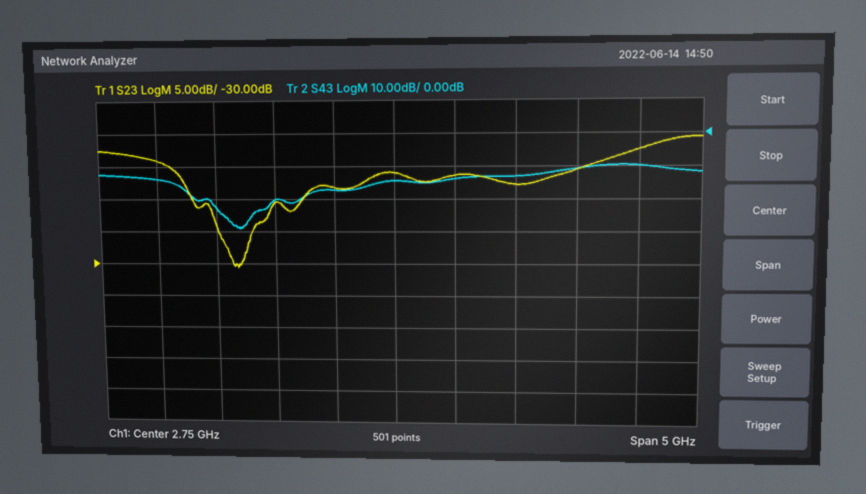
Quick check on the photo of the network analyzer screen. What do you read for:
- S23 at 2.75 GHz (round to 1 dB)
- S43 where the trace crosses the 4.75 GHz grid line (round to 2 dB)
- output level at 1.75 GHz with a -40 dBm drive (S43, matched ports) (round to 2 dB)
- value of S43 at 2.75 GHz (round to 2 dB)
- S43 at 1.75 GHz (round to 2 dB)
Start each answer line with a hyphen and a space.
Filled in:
- -16 dB
- -10 dB
- -60 dBm
- -14 dB
- -20 dB
